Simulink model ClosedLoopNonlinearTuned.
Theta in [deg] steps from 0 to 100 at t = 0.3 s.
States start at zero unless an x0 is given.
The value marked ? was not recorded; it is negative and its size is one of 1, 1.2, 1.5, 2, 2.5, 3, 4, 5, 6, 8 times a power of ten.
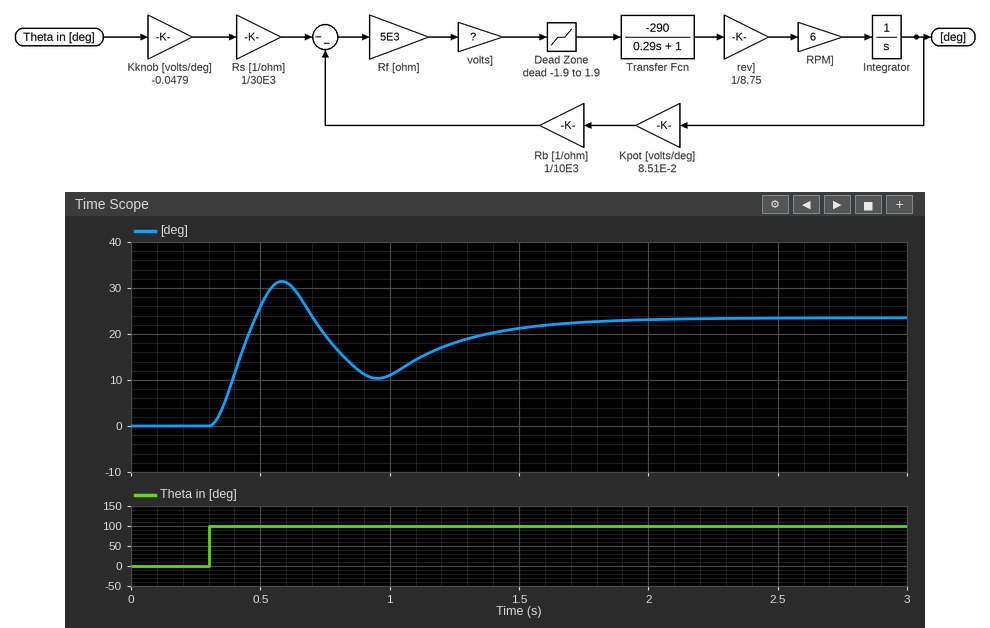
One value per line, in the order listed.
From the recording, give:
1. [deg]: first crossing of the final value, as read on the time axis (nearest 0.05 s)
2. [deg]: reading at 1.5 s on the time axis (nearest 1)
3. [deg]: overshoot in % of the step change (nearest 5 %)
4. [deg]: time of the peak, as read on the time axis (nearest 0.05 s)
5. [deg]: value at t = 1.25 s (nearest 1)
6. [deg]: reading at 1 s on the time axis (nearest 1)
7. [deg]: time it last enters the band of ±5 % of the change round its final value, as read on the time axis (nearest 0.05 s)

0.50 s
21
35 %
0.60 s
18
11
1.70 s
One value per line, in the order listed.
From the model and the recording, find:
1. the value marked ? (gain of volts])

-8
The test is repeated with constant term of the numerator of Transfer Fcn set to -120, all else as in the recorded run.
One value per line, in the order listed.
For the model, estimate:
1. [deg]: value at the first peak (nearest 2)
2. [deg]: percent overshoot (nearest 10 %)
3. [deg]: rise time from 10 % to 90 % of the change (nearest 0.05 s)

28
90 %
0.15 s
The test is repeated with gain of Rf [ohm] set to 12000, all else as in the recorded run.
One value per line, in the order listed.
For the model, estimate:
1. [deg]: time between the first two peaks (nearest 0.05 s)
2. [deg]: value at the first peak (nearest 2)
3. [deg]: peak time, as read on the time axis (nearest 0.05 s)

0.30 s
34
0.45 s
